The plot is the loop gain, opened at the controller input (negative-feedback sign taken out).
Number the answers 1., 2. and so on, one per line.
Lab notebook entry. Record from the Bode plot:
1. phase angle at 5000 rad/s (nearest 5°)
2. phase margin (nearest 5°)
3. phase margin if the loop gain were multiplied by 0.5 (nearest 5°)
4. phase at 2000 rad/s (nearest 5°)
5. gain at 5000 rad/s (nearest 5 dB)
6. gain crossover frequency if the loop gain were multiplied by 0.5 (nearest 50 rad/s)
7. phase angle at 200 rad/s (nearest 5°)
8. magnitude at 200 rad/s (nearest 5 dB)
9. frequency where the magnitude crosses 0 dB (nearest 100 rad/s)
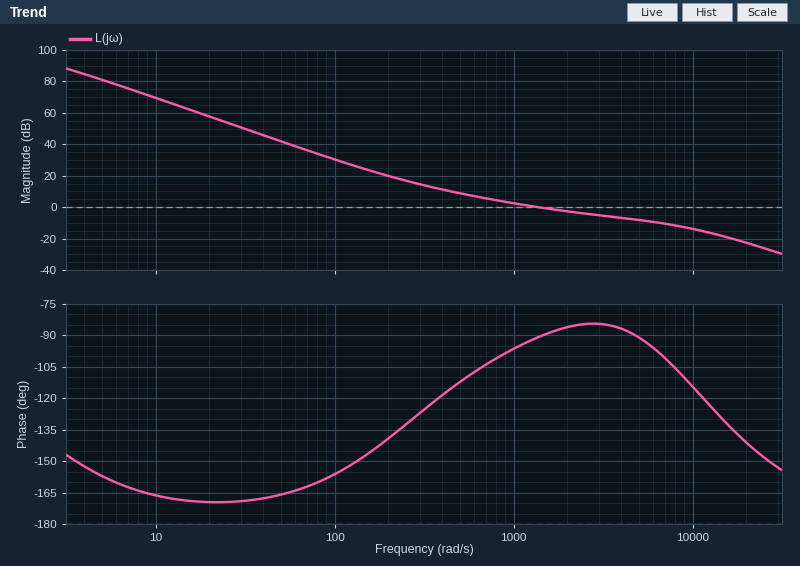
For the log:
1. -90°
2. 90°
3. 75°
4. -85°
5. -10 dB
6. 650 rad/s
7. -140°
8. 20 dB
9. 1400 rad/s
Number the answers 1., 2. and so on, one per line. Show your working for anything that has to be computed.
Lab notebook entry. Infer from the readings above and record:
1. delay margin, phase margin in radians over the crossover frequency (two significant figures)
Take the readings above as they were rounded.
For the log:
1. 90 × π / 180 / 1400 = 0.0011 s
